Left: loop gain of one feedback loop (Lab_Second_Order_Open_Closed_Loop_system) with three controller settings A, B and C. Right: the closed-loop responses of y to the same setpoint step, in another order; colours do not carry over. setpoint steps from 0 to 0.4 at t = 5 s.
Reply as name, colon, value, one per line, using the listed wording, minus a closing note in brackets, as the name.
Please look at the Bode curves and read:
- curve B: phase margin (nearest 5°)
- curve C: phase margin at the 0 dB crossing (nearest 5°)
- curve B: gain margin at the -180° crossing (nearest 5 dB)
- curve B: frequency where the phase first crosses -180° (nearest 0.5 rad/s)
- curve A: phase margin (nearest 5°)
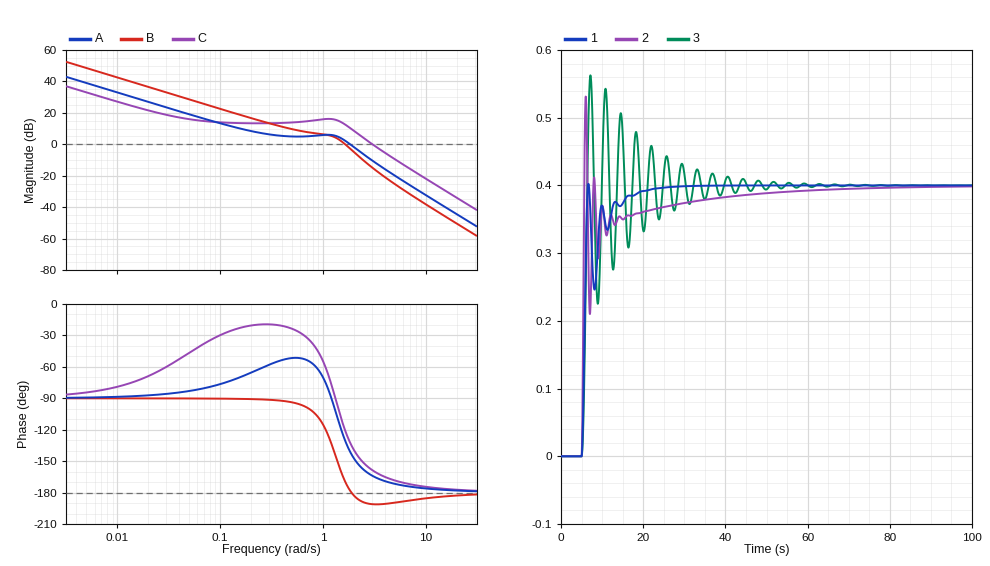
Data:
curve B: phase margin: 10°
curve C: phase margin at the 0 dB crossing: 20°
curve B: gain margin at the -180° crossing: 5 dB
curve B: frequency where the phase first crosses -180°: 2.0 rad/s
curve A: phase margin: 40°
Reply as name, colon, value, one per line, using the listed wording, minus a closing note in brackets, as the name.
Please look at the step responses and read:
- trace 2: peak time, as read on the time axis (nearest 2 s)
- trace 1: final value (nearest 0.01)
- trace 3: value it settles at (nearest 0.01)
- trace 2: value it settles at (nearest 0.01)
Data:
trace 2: peak time, as read on the time axis: 6 s
trace 1: final value: 0.40
trace 3: value it settles at: 0.40
trace 2: value it settles at: 0.40
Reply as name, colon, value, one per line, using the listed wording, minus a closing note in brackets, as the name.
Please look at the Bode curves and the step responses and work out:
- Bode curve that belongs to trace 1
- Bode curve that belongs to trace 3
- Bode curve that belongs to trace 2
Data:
Bode curve that belongs to trace 1: A
Bode curve that belongs to trace 3: B
Bode curve that belongs to trace 2: C
